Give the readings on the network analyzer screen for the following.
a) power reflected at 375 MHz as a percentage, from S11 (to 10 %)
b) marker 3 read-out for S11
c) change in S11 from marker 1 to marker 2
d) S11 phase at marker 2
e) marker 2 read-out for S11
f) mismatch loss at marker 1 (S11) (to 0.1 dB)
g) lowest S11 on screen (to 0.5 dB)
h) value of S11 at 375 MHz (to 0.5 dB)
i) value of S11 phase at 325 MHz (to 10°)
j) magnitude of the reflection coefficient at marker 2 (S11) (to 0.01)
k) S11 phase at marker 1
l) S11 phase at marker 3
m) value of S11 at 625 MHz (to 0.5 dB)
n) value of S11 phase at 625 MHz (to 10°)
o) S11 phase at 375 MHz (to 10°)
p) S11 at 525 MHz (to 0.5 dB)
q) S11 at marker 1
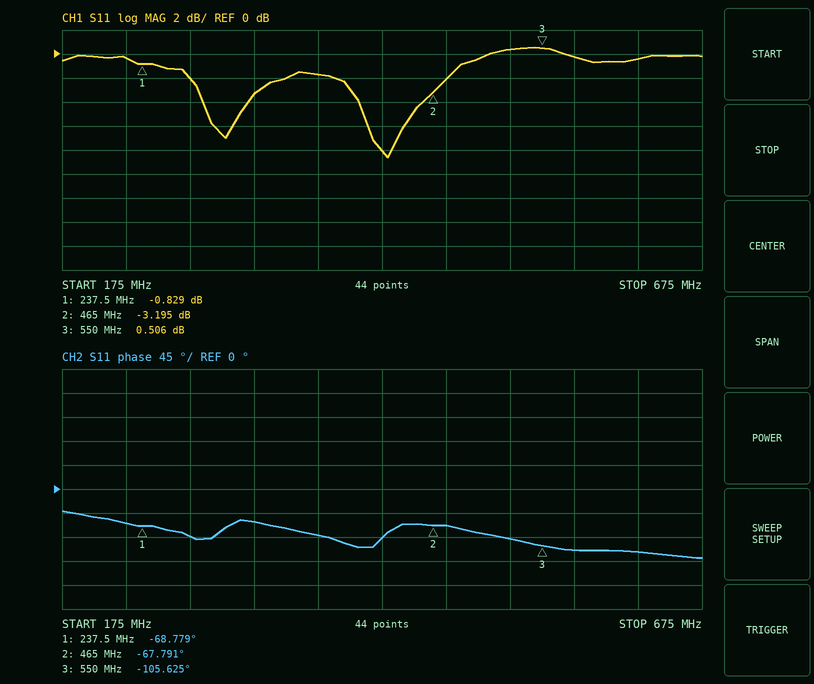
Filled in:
70 %
0.506 dB
-2.366 dB
-67.791°
-3.195 dB
7.6 dB
-8.5 dB
-1.5 dB
-60°
0.69
-68.779°
-105.625°
-0.5 dB
-120°
-90°
0.5 dB
-0.829 dB
